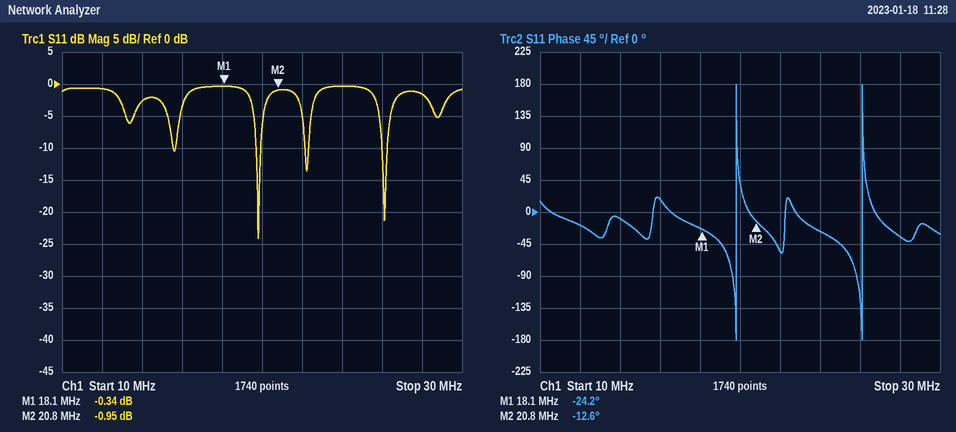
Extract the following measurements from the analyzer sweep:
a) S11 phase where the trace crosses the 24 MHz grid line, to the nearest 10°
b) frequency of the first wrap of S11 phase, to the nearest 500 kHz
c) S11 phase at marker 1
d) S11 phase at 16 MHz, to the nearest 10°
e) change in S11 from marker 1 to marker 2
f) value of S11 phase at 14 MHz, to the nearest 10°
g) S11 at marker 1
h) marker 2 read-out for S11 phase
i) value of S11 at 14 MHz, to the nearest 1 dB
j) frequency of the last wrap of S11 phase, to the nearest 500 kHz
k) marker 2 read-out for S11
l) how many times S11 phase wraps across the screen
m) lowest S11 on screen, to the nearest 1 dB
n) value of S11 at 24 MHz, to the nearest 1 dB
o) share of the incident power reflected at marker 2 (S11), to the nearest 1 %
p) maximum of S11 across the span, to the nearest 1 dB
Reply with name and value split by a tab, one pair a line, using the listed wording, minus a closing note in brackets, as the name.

S11 phase where the trace crosses the 24 MHz grid line, to the nearest 10°	-30°
frequency of the first wrap of S11 phase, to the nearest 500 kHz	20.0 MHz
S11 phase at marker 1	-24.2°
S11 phase at 16 MHz, to the nearest 10°	20°
change in S11 from marker 1 to marker 2	-0.61 dB
value of S11 phase at 14 MHz, to the nearest 10°	-10°
S11 at marker 1	-0.34 dB
marker 2 read-out for S11 phase	-12.6°
value of S11 at 14 MHz, to the nearest 1 dB	-3 dB
frequency of the last wrap of S11 phase, to the nearest 500 kHz	26.0 MHz
marker 2 read-out for S11	-0.95 dB
how many times S11 phase wraps across the screen	2
lowest S11 on screen, to the nearest 1 dB	-24 dB
value of S11 at 24 MHz, to the nearest 1 dB	0 dB
share of the incident power reflected at marker 2 (S11), to the nearest 1 %	80 %
maximum of S11 across the span, to the nearest 1 dB	0 dB
